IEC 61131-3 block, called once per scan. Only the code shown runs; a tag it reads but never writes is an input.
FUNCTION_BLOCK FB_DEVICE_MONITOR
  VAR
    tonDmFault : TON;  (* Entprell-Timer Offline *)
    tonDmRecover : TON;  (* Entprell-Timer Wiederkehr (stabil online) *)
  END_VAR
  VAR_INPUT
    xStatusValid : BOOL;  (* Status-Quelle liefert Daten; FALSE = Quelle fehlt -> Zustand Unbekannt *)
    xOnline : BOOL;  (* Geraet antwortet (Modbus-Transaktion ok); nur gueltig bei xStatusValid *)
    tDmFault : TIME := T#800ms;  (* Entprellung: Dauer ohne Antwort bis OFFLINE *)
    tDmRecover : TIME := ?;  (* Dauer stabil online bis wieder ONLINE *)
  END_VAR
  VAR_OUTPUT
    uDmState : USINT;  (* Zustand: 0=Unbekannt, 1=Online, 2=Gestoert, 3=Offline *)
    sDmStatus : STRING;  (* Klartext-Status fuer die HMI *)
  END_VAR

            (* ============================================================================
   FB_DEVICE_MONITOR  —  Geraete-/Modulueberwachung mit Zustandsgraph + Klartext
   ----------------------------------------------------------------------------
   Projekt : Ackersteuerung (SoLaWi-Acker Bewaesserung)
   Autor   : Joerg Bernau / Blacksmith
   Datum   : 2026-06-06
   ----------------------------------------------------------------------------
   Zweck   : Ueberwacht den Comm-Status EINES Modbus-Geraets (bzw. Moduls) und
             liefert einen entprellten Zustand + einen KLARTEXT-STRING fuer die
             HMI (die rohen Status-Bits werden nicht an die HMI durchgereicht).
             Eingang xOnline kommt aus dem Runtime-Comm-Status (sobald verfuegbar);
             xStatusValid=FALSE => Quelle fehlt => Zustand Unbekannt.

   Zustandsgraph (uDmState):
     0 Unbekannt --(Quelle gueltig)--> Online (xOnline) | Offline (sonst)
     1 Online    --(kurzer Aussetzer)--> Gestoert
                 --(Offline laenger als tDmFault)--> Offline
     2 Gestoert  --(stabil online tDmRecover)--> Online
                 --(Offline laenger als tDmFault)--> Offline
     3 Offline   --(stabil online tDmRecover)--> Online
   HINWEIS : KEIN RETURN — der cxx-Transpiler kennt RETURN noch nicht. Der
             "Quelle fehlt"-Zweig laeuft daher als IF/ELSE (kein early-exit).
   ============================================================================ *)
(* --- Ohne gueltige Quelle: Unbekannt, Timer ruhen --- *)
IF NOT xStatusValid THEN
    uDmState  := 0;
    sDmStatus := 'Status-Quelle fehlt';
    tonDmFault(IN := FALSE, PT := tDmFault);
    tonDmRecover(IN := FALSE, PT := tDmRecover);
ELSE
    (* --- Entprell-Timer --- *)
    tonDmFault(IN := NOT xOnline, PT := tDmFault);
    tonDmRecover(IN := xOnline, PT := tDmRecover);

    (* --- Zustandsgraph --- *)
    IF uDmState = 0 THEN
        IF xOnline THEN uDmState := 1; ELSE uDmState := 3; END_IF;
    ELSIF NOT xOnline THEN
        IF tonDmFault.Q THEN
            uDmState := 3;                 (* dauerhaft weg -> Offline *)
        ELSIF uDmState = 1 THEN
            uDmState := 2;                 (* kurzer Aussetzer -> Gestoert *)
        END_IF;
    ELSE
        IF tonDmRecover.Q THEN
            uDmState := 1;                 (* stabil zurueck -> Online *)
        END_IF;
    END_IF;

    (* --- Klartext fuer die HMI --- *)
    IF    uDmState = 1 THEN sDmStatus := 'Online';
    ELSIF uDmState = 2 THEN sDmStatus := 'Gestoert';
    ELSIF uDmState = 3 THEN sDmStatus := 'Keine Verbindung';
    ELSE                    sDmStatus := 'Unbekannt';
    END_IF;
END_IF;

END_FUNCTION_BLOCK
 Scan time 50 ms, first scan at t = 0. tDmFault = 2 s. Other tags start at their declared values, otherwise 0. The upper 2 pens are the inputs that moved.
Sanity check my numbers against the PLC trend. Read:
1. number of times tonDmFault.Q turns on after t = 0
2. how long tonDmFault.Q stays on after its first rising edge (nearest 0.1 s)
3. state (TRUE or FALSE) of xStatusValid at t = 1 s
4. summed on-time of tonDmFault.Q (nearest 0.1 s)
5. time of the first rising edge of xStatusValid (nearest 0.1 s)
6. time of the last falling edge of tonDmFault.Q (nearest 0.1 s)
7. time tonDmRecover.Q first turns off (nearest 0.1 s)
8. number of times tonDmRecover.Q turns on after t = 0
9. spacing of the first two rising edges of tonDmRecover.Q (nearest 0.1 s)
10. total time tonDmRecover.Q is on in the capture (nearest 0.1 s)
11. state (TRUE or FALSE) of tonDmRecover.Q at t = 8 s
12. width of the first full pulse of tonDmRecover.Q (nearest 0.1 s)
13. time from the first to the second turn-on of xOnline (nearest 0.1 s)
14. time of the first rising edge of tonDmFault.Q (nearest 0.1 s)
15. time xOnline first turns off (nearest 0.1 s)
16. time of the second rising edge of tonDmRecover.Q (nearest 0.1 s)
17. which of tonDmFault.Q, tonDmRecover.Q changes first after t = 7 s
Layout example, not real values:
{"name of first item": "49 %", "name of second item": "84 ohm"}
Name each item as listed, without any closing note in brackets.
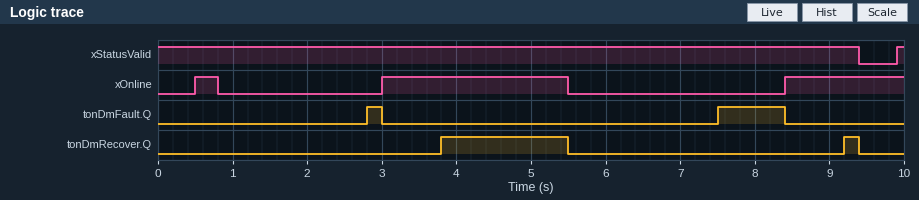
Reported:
{"number of times tonDmFault.Q turns on after t = 0": "2", "how long tonDmFault.Q stays on after its first rising edge": "0.2 s", "state (TRUE or FALSE) of xStatusValid at t = 1 s": "TRUE", "summed on-time of tonDmFault.Q": "1.1 s", "time of the first rising edge of xStatusValid": "9.9 s", "time of the last falling edge of tonDmFault.Q": "8.4 s", "time tonDmRecover.Q first turns off": "5.5 s", "number of times tonDmRecover.Q turns on after t = 0": "2", "spacing of the first two rising edges of tonDmRecover.Q": "5.4 s", "total time tonDmRecover.Q is on in the capture": "1.9 s", "state (TRUE or FALSE) of tonDmRecover.Q at t = 8 s": "FALSE", "width of the first full pulse of tonDmRecover.Q": "1.7 s", "time from the first to the second turn-on of xOnline": "2.5 s", "time of the first rising edge of tonDmFault.Q": "2.8 s", "time xOnline first turns off": "0.8 s", "time of the second rising edge of tonDmRecover.Q": "9.2 s", "which of tonDmFault.Q, tonDmRecover.Q changes first after t = 7 s": "tonDmFault.Q"}
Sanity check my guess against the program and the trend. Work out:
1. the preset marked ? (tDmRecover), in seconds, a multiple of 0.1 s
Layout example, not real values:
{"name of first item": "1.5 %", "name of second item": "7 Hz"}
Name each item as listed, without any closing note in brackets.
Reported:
{"the preset marked ? (tDmRecover), in seconds, a multiple of 0.1 s": "0.8 s"}
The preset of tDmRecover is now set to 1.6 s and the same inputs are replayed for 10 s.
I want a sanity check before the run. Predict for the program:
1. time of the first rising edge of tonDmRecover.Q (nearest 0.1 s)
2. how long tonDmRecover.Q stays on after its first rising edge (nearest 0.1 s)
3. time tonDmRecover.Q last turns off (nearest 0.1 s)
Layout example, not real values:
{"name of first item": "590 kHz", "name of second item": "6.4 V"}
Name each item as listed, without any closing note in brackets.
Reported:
{"time of the first rising edge of tonDmRecover.Q": "4.6 s", "how long tonDmRecover.Q stays on after its first rising edge": "0.9 s", "time tonDmRecover.Q last turns off": "5.5 s"}
